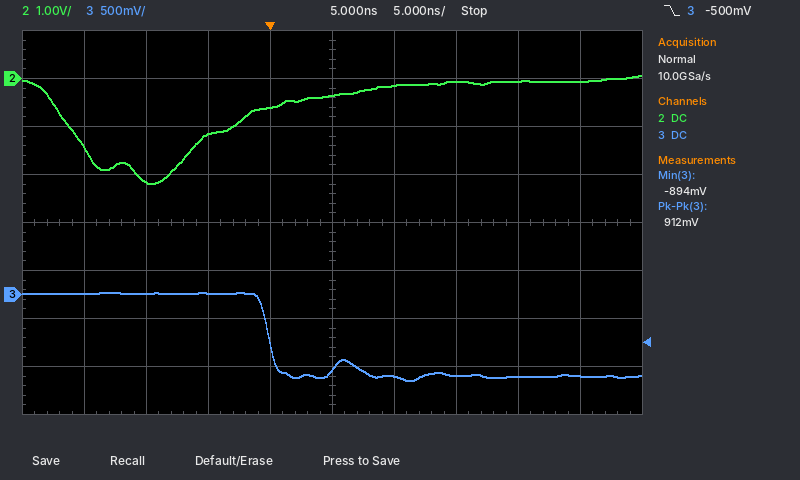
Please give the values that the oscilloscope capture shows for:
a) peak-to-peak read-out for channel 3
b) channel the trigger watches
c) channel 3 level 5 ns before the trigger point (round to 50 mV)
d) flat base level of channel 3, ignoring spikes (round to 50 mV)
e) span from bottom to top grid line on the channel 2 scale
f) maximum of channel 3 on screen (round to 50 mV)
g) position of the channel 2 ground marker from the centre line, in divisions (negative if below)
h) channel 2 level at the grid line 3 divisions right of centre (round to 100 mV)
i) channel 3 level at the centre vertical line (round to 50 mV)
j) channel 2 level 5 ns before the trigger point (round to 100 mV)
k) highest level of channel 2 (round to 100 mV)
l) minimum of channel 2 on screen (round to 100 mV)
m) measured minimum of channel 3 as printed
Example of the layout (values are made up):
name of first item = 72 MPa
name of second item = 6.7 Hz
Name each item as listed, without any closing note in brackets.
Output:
peak-to-peak read-out for channel 3 = 912 mV
channel the trigger watches = channel 3
channel 3 level 5 ns before the trigger point = 0 mV
flat base level of channel 3, ignoring spikes = -850 mV
span from bottom to top grid line on the channel 2 scale = 8 V
maximum of channel 3 on screen = 0 mV
position of the channel 2 ground marker from the centre line, in divisions = +3.0 div
channel 2 level at the grid line 3 divisions right of centre = -100 mV
channel 3 level at the centre vertical line = -800 mV
channel 2 level 5 ns before the trigger point = -1.2 V
highest level of channel 2 = 100 mV
minimum of channel 2 on screen = -2.2 V
measured minimum of channel 3 as printed = -894 mV
